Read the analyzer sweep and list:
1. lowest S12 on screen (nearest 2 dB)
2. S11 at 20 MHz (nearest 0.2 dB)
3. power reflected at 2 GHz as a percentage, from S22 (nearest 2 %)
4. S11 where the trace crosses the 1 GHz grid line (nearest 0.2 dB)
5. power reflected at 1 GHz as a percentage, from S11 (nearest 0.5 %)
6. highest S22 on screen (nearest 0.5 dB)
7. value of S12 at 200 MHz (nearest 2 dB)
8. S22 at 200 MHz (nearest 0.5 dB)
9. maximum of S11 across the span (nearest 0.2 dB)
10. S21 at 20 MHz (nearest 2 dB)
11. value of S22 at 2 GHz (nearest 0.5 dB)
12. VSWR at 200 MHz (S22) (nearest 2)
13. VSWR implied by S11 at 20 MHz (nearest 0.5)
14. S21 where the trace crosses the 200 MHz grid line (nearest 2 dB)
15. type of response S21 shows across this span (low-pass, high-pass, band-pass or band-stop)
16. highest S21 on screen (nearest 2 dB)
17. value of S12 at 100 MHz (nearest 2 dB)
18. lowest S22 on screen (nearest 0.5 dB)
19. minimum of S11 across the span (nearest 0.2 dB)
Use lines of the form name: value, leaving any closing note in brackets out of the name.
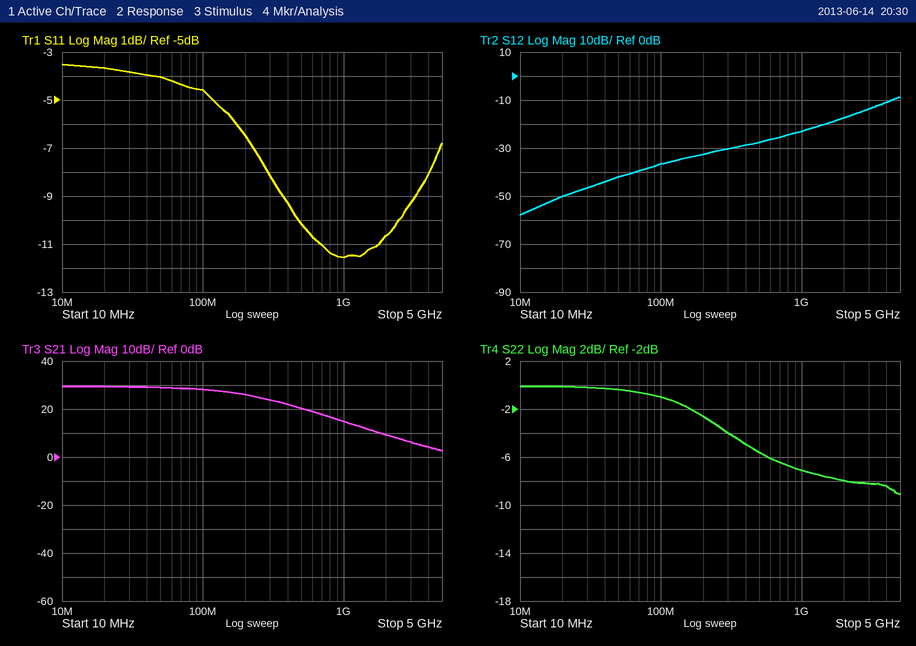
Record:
lowest S12 on screen: -58 dB
S11 at 20 MHz: -3.6 dB
power reflected at 2 GHz as a percentage, from S22: 16 %
S11 where the trace crosses the 1 GHz grid line: -11.6 dB
power reflected at 1 GHz as a percentage, from S11: 7.0 %
highest S22 on screen: 0.0 dB
value of S12 at 200 MHz: -32 dB
S22 at 200 MHz: -2.5 dB
maximum of S11 across the span: -3.6 dB
S21 at 20 MHz: 30 dB
value of S22 at 2 GHz: -8.0 dB
VSWR at 200 MHz (S22): 6
VSWR implied by S11 at 20 MHz: 5.0
S21 where the trace crosses the 200 MHz grid line: 26 dB
type of response S21 shows across this span: low-pass
highest S21 on screen: 30 dB
value of S12 at 100 MHz: -36 dB
lowest S22 on screen: -9.0 dB
minimum of S11 across the span: -11.6 dB
